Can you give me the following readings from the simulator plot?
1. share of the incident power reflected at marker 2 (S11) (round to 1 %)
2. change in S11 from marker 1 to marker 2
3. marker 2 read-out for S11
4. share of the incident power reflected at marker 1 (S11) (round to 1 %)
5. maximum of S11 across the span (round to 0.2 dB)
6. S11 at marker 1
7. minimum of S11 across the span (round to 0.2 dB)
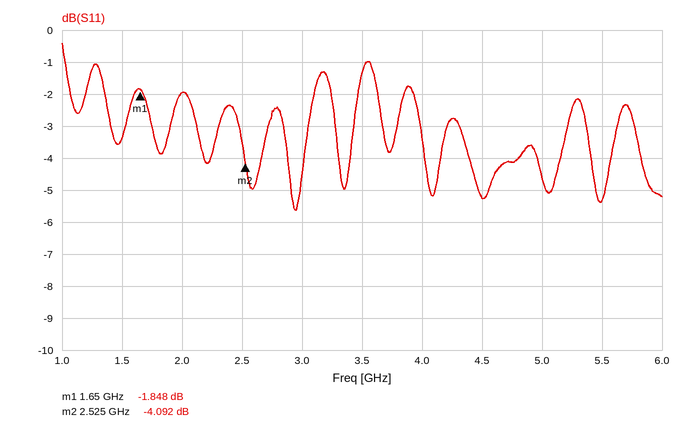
39 %
-2.244 dB
-4.092 dB
65 %
-0.4 dB
-1.848 dB
-5.6 dB
